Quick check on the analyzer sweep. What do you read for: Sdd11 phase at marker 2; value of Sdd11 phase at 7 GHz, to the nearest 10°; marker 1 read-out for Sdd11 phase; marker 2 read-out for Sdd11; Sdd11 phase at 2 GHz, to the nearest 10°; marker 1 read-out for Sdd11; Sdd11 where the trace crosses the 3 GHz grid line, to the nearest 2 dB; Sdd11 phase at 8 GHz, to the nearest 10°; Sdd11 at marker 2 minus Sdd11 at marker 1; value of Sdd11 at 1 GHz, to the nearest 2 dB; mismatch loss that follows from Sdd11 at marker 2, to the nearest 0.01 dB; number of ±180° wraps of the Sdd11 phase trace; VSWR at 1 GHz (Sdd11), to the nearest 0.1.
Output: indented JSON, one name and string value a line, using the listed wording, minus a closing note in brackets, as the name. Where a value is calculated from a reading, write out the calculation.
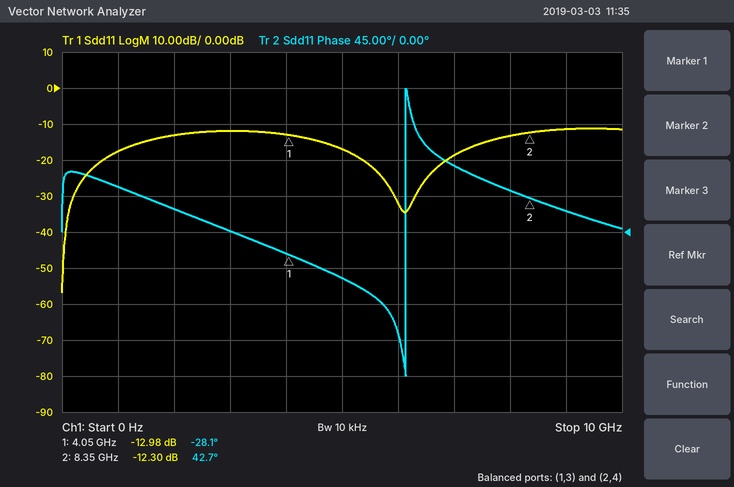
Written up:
{
  "Sdd11 phase at marker 2": "42.7°",
  "value of Sdd11 phase at 7 GHz, to the nearest 10°": "80°",
  "marker 1 read-out for Sdd11 phase": "-28.1°",
  "marker 2 read-out for Sdd11": "-12.30 dB",
  "Sdd11 phase at 2 GHz, to the nearest 10°": "30°",
  "marker 1 read-out for Sdd11": "-12.98 dB",
  "Sdd11 where the trace crosses the 3 GHz grid line, to the nearest 2 dB": "-12 dB",
  "Sdd11 phase at 8 GHz, to the nearest 10°": "50°",
  "Sdd11 at marker 2 minus Sdd11 at marker 1": "-12.3 − (-12.98) = 0.68 dB",
  "value of Sdd11 at 1 GHz, to the nearest 2 dB": "-18 dB",
  "mismatch loss that follows from Sdd11 at marker 2, to the nearest 0.01 dB": "−10 log10(1 − 10^(-12.3/10)) ≈ 0.26 dB",
  "number of ±180° wraps of the Sdd11 phase trace": "1",
  "VSWR at 1 GHz (Sdd11), to the nearest 0.1": "|Γ| = 10^(-18/20) = 0.1259; VSWR = (1 + 0.1259)/(1 − 0.1259) ≈ 1.3"
}
